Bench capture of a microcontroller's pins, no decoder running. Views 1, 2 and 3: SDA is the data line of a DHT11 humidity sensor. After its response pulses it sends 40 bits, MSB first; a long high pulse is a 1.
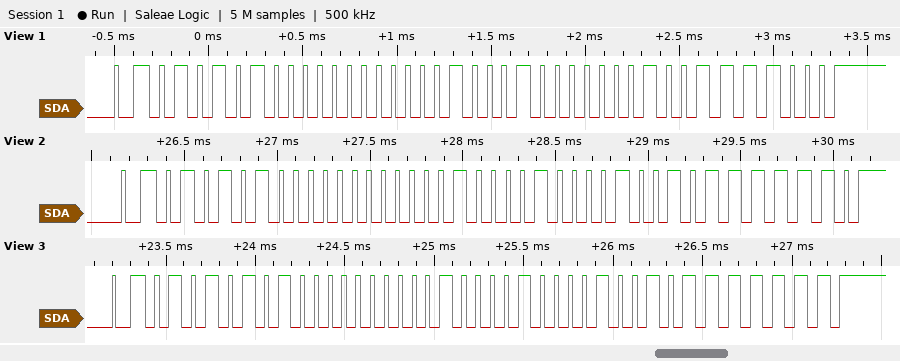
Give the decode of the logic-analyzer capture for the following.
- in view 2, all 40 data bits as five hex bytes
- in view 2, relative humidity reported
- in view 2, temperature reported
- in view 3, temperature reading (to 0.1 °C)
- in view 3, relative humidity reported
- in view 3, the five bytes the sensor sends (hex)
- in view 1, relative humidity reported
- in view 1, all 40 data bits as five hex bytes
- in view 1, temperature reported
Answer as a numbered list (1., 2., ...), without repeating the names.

1. 54 00 21 09 7E
2. 84 %
3. 33.9 °C
4. 33.9 °C
5. 85 %
6. 55 00 21 09 7F
7. 84 %
8. 54 00 22 02 78
9. 34.2 °C
